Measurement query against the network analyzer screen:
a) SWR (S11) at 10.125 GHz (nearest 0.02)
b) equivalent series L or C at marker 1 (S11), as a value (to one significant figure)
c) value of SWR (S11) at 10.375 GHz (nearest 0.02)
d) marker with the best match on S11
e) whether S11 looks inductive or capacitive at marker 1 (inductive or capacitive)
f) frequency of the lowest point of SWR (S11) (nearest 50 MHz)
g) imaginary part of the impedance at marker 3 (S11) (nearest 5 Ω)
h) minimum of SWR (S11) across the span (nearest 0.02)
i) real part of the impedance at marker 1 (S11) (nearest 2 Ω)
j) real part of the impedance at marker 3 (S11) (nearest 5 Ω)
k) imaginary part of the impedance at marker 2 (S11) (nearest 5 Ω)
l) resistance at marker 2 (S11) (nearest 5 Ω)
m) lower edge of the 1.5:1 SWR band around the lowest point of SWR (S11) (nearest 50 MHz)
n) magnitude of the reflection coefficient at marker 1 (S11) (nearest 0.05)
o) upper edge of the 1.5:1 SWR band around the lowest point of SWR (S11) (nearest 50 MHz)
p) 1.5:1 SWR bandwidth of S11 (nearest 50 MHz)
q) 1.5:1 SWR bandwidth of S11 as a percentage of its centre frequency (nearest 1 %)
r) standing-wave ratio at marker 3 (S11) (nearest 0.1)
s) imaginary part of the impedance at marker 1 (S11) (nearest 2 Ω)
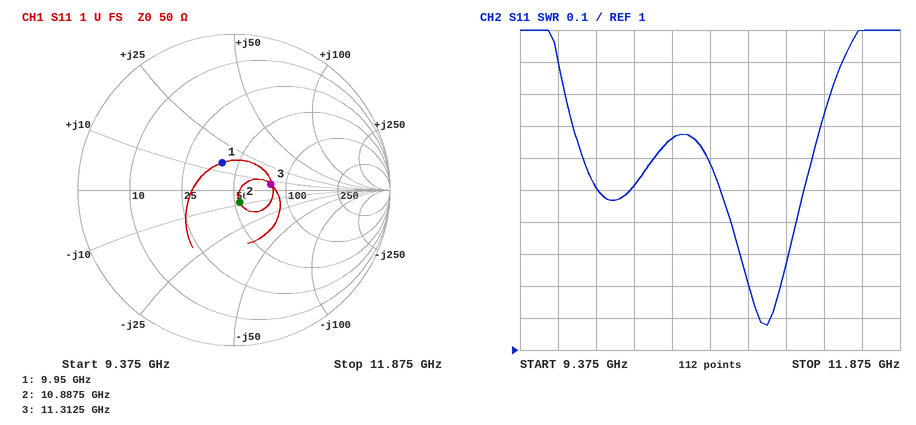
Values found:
1.52
200 pH
1.66
marker 2
inductive
11.00 GHz
+5 Ω
1.08
40 Ω
80 Ω
-10 Ω
55 Ω
10.70 GHz
0.20
11.25 GHz
550 MHz
5 %
1.6
+14 Ω
